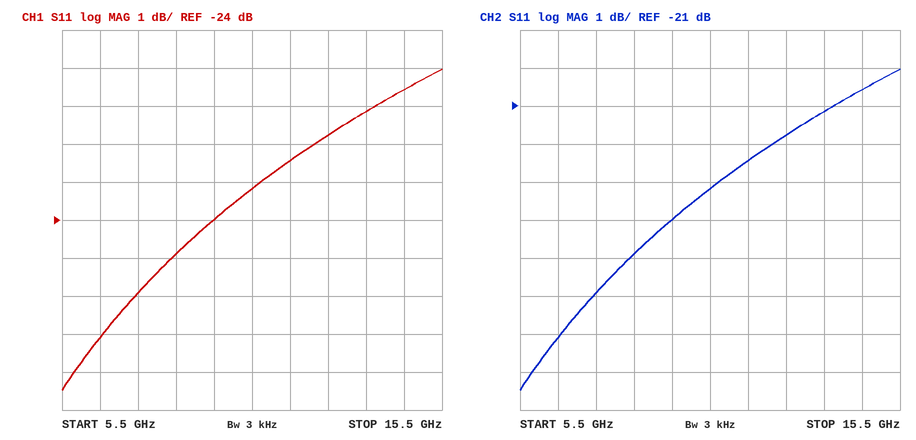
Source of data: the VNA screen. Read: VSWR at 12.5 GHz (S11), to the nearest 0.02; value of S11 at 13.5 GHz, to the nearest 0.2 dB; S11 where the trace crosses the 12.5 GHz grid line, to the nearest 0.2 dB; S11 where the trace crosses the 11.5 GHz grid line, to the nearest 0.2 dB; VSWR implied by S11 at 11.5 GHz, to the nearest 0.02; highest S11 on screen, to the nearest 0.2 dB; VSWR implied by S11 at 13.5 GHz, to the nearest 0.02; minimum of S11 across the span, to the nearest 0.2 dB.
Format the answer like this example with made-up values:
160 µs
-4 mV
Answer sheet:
1.18
-21.2 dB
-21.8 dB
-22.4 dB
1.16
-20.0 dB
1.20
-28.4 dB
